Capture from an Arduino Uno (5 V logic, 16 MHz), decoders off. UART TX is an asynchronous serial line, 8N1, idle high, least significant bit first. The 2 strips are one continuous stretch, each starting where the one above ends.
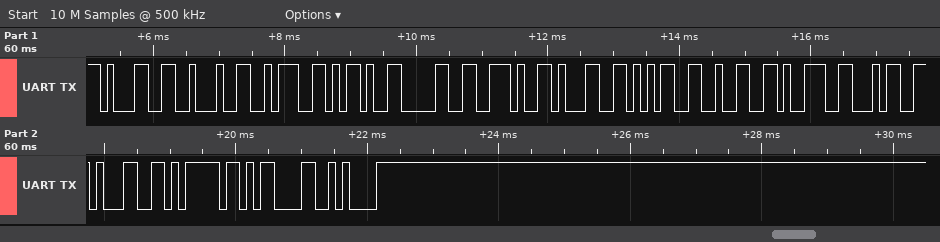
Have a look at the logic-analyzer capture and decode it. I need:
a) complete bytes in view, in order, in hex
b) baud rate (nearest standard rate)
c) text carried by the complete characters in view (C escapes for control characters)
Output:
31 22 3A 2D 30 2E 31 35 32 39 34 31 7D 0D 0A
9600 baud
"1\":-0.152941}\r\n"
